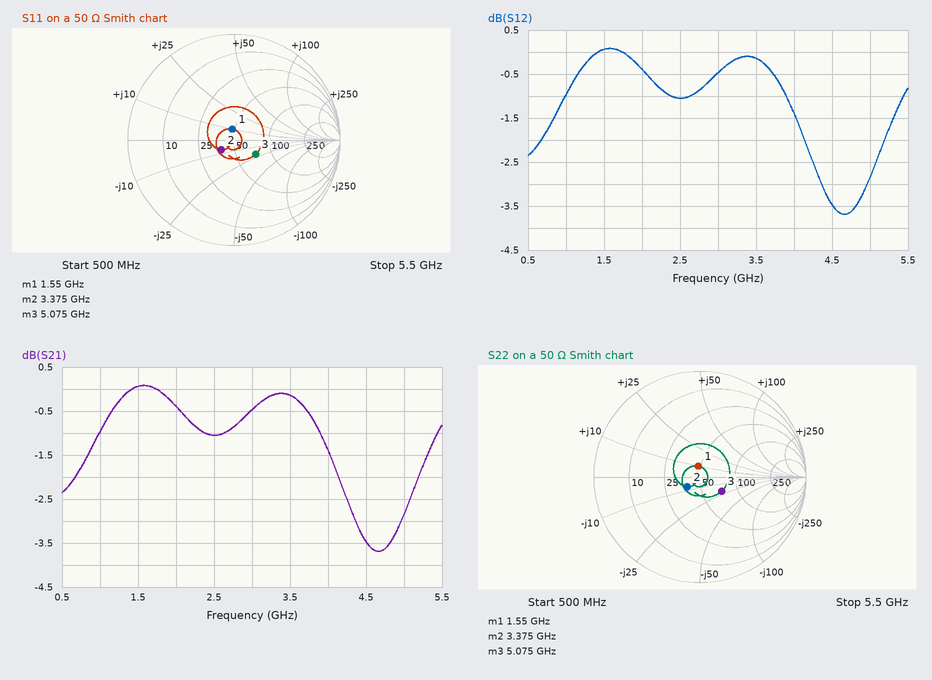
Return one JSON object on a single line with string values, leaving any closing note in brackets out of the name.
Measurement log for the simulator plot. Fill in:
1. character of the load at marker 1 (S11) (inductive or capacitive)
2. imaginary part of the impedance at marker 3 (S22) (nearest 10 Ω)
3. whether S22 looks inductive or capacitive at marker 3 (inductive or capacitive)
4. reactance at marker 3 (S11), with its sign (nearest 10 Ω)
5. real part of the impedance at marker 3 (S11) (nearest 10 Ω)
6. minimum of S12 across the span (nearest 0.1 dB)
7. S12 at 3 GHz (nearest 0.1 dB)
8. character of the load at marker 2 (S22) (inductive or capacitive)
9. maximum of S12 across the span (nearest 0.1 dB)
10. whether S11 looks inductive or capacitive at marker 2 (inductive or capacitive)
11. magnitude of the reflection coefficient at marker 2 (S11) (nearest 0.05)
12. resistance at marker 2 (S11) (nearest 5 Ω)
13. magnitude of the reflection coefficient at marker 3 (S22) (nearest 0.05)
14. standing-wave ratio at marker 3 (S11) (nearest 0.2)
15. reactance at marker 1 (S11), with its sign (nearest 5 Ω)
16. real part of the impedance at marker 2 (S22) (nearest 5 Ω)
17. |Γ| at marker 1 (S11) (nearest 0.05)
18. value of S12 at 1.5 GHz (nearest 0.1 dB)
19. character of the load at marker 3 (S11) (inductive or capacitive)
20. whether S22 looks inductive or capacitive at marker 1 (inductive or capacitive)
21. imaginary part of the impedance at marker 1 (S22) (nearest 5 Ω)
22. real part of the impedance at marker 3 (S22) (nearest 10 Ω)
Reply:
{"character of the load at marker 1 (S11)": "inductive", "imaginary part of the impedance at marker 3 (S22)": "-20 Ω", "whether S22 looks inductive or capacitive at marker 3": "capacitive", "reactance at marker 3 (S11), with its sign": "-20 Ω", "real part of the impedance at marker 3 (S11)": "70 Ω", "minimum of S12 across the span": "-3.7 dB", "S12 at 3 GHz": "-0.5 dB", "character of the load at marker 2 (S22)": "capacitive", "maximum of S12 across the span": "0.1 dB", "whether S11 looks inductive or capacitive at marker 2": "capacitive", "magnitude of the reflection coefficient at marker 2 (S11)": "0.15", "resistance at marker 2 (S11)": "40 Ω", "magnitude of the reflection coefficient at marker 3 (S22)": "0.25", "standing-wave ratio at marker 3 (S11)": "1.6", "reactance at marker 1 (S11), with its sign": "+10 Ω", "real part of the impedance at marker 2 (S22)": "40 Ω", "|Γ| at marker 1 (S11)": "0.10", "value of S12 at 1.5 GHz": "0.1 dB", "character of the load at marker 3 (S11)": "capacitive", "whether S22 looks inductive or capacitive at marker 1": "inductive", "imaginary part of the impedance at marker 1 (S22)": "+10 Ω", "real part of the impedance at marker 3 (S22)": "70 Ω"}
